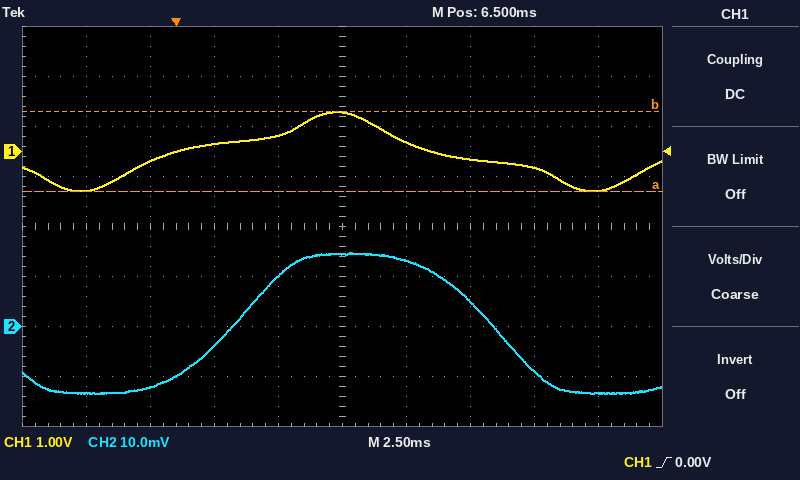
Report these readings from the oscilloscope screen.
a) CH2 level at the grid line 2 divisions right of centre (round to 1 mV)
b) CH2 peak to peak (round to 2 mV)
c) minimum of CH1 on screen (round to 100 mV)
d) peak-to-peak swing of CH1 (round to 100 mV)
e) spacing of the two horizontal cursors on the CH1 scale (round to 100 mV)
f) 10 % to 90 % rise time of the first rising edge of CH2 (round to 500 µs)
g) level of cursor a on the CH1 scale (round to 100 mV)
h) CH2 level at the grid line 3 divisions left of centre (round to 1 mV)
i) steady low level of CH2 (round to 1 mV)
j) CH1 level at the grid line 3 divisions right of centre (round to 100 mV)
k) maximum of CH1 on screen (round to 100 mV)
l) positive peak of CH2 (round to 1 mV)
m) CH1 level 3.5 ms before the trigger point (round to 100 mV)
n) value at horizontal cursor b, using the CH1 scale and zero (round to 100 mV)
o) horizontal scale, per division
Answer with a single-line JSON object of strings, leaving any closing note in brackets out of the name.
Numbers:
{"CH2 level at the grid line 2 divisions right of centre": "5 mV", "CH2 peak to peak": "28 mV", "minimum of CH1 on screen": "-800 mV", "peak-to-peak swing of CH1": "1.6 V", "spacing of the two horizontal cursors on the CH1 scale": "1.6 V", "10 % to 90 % rise time of the first rising edge of CH2": "4.5 ms", "level of cursor a on the CH1 scale": "-800 mV", "CH2 level at the grid line 3 divisions left of centre": "-12 mV", "steady low level of CH2": "-13 mV", "CH1 level at the grid line 3 divisions right of centre": "-300 mV", "maximum of CH1 on screen": "800 mV", "positive peak of CH2": "15 mV", "CH1 level 3.5 ms before the trigger point": "-800 mV", "value at horizontal cursor b, using the CH1 scale and zero": "800 mV", "horizontal scale, per division": "2.5 ms"}
